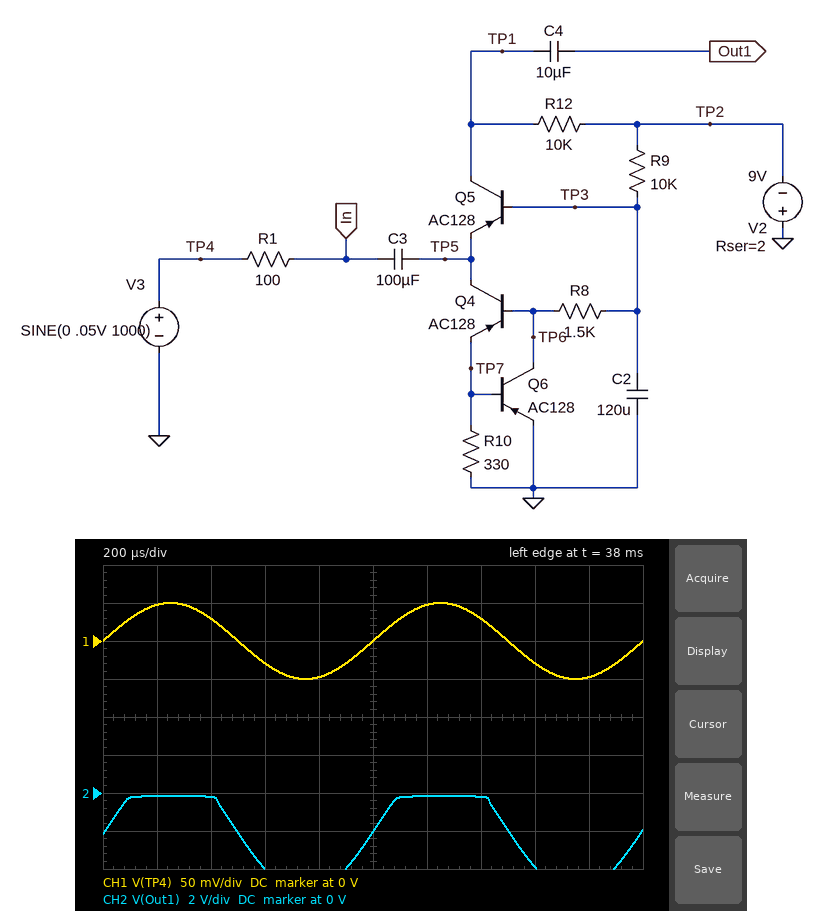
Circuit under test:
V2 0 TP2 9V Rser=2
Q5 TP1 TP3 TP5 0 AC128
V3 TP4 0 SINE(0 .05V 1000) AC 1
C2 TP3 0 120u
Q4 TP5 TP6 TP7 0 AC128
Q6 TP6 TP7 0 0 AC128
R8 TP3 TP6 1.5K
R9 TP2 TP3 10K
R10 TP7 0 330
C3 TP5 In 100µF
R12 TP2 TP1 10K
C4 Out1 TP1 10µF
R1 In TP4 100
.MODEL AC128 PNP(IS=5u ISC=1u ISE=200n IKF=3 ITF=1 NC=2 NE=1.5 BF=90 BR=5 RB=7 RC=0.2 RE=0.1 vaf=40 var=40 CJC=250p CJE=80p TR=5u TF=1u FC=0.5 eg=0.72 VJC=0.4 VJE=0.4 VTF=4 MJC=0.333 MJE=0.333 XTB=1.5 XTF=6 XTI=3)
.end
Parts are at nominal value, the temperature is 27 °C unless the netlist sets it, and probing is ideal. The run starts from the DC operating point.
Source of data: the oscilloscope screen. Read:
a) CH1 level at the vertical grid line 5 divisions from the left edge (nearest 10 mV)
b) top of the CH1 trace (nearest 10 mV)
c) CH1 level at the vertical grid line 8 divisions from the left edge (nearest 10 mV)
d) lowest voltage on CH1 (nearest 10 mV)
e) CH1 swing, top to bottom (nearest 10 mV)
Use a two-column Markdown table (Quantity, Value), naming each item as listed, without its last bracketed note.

| Quantity | Value |
|---|---|
| CH1 level at the vertical grid line 5 divisions from the left edge | 0 V |
| top of the CH1 trace | 50 mV |
| CH1 level at the vertical grid line 8 divisions from the left edge | -30 mV |
| lowest voltage on CH1 | -50 mV |
| CH1 swing, top to bottom | 100 mV |
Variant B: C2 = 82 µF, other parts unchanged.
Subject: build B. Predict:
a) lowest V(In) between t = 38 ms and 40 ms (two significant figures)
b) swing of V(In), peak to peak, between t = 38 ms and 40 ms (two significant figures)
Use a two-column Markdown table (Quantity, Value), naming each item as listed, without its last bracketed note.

| Quantity | Value |
|---|---|
| lowest V(In) between t = 38 ms and 40 ms | -89 mV |
| swing of V(In), peak to peak, between t = 38 ms and 40 ms | 41 mV |
